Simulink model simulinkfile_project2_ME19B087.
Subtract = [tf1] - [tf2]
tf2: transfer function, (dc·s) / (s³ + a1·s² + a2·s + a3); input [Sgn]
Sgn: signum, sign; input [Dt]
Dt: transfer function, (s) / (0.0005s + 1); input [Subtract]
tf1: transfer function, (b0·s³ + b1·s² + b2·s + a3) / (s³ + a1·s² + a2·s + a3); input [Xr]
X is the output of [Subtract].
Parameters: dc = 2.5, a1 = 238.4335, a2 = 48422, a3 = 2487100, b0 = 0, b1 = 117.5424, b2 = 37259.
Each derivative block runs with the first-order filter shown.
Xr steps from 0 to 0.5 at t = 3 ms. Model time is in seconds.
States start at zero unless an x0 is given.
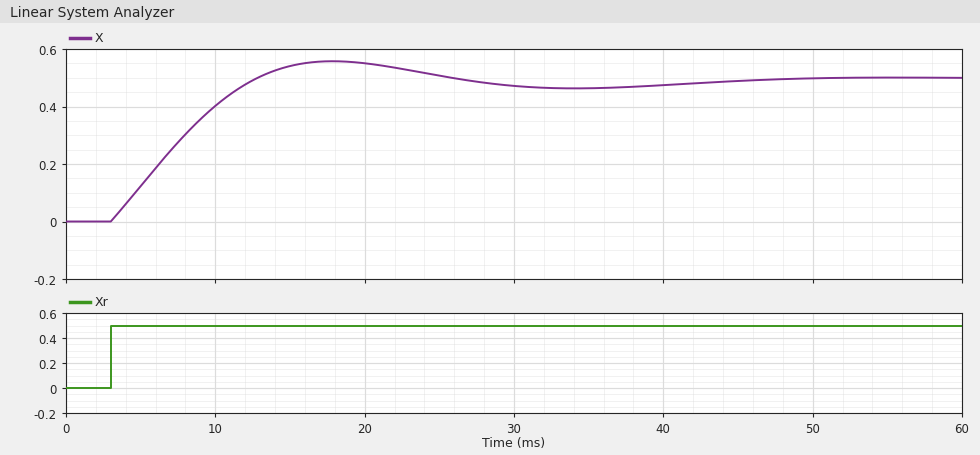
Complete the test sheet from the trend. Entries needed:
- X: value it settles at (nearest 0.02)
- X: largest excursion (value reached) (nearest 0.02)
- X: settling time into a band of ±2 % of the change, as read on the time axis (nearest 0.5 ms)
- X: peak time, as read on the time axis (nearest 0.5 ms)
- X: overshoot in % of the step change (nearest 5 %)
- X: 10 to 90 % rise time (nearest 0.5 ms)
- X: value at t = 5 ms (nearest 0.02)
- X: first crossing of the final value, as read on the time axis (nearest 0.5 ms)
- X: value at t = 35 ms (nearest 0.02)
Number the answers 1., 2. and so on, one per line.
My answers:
1. 0.50
2. 0.56
3. 45.5 ms
4. 18.0 ms
5. 10 %
6. 7.5 ms
7. 0.12
8. 13.0 ms
9. 0.46
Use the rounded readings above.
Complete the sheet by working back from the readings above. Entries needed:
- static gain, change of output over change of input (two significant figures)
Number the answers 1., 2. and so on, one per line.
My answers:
1. 1.0
